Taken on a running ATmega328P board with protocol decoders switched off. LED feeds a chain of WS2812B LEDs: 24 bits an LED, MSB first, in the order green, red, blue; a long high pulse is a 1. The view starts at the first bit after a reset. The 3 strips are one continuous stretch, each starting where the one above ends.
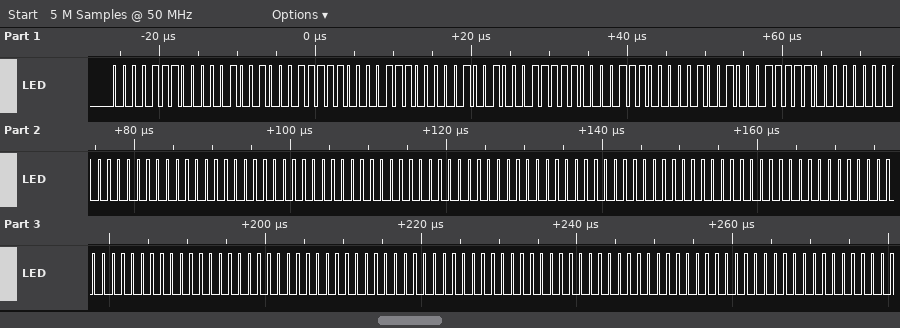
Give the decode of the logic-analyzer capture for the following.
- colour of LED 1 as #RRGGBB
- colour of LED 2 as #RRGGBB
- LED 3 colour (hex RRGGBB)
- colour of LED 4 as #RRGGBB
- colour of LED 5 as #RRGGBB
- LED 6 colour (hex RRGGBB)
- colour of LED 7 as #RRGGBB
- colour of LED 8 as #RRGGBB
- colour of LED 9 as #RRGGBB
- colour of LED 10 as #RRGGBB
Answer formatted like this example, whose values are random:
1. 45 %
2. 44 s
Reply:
1. #090E1F
2. #090E1F
3. #090E1F
4. #000000
5. #000000
6. #000000
7. #000000
8. #000000
9. #000000
10. #000000
